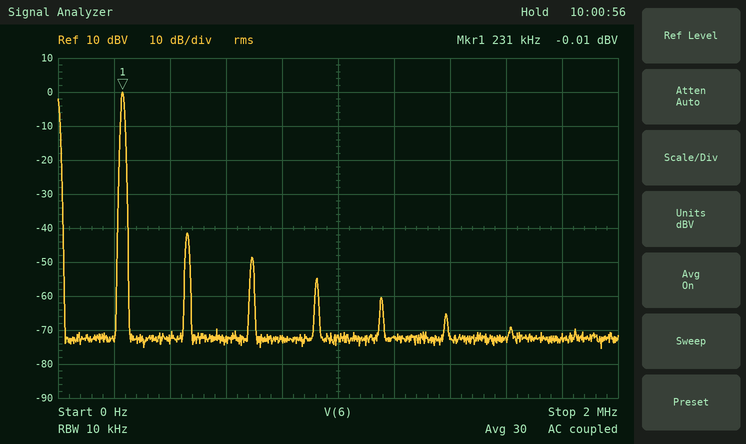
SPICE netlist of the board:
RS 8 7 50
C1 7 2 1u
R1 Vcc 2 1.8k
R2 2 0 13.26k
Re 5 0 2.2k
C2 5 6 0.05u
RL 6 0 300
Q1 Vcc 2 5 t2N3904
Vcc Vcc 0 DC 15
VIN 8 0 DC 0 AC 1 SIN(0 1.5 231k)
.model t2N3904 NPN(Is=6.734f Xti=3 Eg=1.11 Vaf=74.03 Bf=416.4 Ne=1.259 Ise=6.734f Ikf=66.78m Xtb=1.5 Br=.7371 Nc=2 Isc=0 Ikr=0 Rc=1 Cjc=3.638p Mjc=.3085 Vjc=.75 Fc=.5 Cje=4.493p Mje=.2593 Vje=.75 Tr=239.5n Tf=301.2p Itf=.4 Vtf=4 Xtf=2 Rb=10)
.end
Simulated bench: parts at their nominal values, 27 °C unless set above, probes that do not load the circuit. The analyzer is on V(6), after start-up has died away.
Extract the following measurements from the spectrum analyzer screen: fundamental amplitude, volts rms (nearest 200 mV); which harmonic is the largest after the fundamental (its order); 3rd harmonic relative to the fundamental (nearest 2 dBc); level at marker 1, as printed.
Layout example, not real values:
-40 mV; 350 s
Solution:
1.0 V; 2; -48 dBc; -0.01 dBV
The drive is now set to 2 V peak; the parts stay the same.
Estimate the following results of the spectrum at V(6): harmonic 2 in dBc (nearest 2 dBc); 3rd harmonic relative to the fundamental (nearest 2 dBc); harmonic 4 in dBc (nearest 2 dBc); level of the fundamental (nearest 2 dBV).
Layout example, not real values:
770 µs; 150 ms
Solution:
-24 dBc; -26 dBc; -32 dBc; 2 dBV
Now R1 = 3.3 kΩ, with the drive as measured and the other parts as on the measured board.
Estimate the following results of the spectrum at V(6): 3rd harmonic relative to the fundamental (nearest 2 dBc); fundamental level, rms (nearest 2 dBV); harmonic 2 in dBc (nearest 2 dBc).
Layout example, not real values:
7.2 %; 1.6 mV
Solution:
-40 dBc; 0 dBV; -34 dBc
